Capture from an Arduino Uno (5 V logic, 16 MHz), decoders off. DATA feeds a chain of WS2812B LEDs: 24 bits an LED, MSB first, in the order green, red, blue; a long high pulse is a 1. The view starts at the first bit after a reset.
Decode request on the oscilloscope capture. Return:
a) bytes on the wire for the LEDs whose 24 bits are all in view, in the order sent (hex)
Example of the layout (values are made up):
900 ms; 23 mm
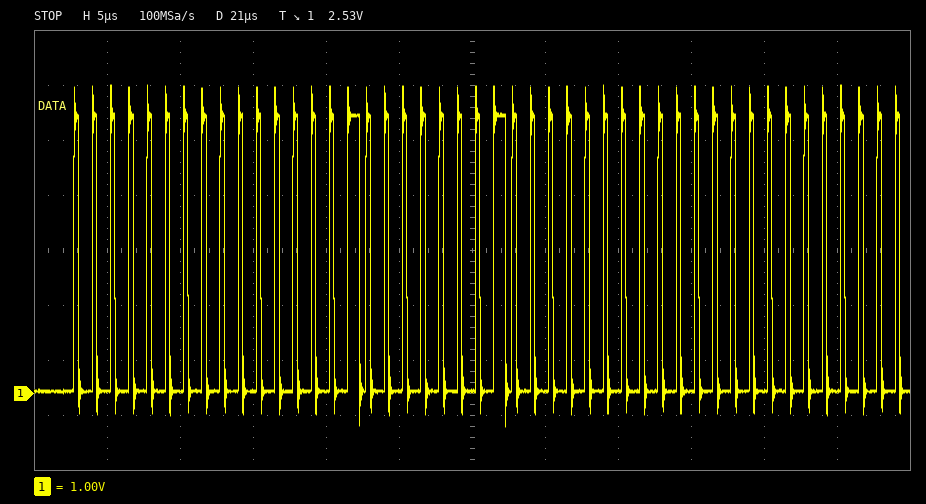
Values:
00 01 01
